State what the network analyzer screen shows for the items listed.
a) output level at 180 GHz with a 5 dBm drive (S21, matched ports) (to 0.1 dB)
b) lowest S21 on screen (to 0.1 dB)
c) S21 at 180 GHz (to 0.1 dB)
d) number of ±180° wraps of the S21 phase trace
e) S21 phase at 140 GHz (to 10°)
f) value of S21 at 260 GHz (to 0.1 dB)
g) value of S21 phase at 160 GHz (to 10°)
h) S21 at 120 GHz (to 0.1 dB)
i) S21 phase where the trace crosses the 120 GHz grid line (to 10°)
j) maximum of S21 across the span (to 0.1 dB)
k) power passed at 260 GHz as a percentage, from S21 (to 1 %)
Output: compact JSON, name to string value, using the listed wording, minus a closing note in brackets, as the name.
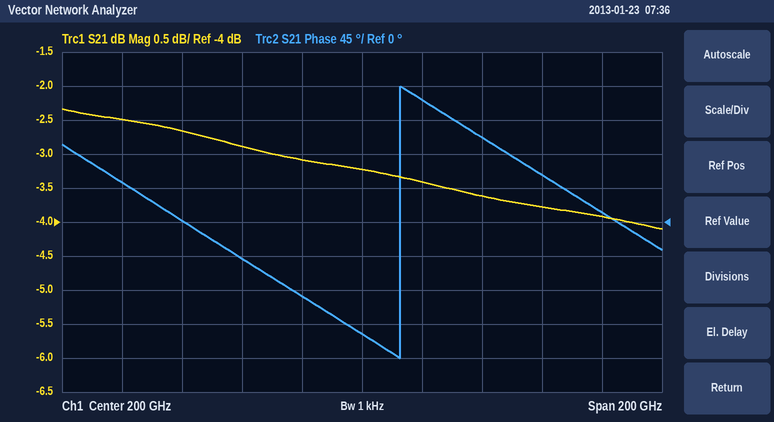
{"output level at 180 GHz with a 5 dBm drive (S21, matched ports)": "1.9 dBm", "lowest S21 on screen": "-4.1 dB", "S21 at 180 GHz": "-3.1 dB", "number of ±180° wraps of the S21 phase trace": "1", "S21 phase at 140 GHz": "0°", "value of S21 at 260 GHz": "-3.8 dB", "value of S21 phase at 160 GHz": "-50°", "S21 at 120 GHz": "-2.5 dB", "S21 phase where the trace crosses the 120 GHz grid line": "50°", "maximum of S21 across the span": "-2.3 dB", "power passed at 260 GHz as a percentage, from S21": "42 %"}
